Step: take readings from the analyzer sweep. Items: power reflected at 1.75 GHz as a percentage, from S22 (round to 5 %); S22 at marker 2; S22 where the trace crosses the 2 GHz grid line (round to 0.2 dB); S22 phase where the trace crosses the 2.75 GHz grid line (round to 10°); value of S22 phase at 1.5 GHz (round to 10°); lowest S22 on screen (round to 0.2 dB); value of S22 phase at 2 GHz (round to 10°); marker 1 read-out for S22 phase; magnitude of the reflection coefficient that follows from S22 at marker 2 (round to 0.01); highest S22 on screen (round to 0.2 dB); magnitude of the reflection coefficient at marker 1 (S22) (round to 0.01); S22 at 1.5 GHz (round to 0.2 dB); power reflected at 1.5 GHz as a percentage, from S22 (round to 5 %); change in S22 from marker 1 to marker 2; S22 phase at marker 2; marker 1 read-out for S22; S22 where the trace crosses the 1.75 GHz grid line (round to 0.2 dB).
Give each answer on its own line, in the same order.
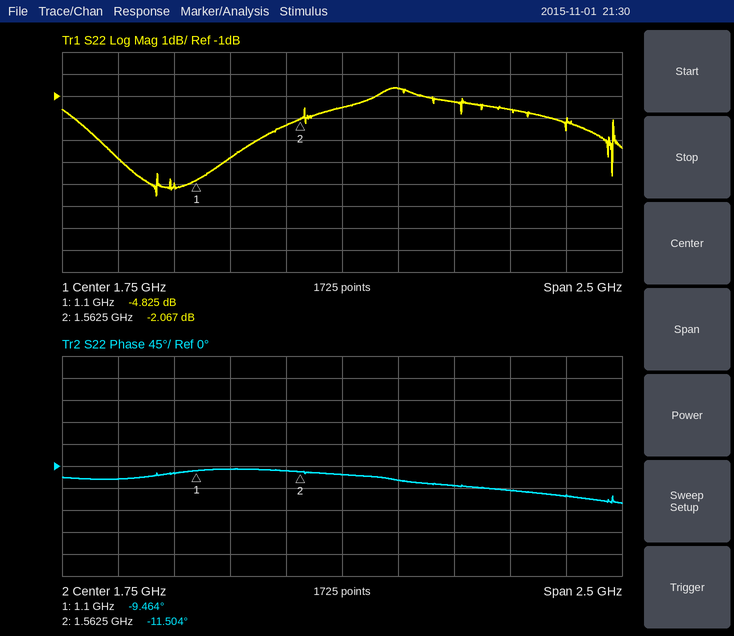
70 %
-2.067 dB
-0.6 dB
-60°
-10°
-5.6 dB
-30°
-9.464°
0.79
-0.6 dB
0.57
-2.4 dB
60 %
2.758 dB
-11.504°
-4.825 dB
-1.6 dB
